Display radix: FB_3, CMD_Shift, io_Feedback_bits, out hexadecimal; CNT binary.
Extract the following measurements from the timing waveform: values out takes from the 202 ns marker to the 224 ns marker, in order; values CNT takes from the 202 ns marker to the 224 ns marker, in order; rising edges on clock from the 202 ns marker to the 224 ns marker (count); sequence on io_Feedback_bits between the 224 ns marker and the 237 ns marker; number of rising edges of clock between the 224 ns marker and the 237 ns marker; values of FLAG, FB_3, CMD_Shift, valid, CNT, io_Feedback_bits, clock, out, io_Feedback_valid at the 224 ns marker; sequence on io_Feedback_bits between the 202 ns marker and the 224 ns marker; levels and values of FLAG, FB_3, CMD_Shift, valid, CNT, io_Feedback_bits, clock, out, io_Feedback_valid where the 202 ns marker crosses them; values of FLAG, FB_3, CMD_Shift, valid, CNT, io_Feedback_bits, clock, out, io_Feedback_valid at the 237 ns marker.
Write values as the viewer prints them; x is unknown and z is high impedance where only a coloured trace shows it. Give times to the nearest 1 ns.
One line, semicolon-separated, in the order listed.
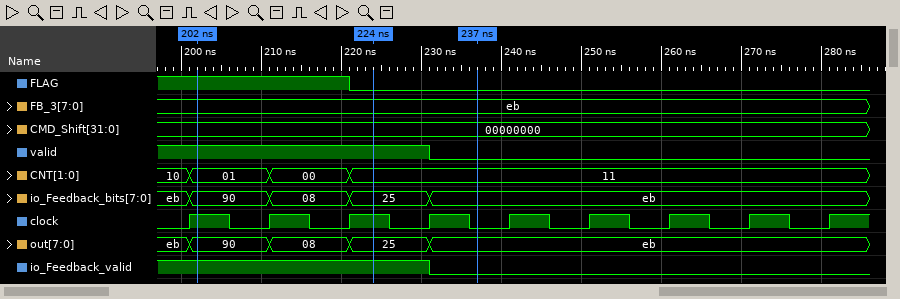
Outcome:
90, 08, 25; 01, 00, 11; 2; 25, eb; 1; FLAG=0, FB_3=eb, CMD_Shift=00000000, valid=1, CNT=11, io_Feedback_bits=25, clock=1, out=25, io_Feedback_valid=1; 90, 08, 25; FLAG=1, FB_3=eb, CMD_Shift=00000000, valid=1, CNT=01, io_Feedback_bits=90, clock=1, out=90, io_Feedback_valid=1; FLAG=0, FB_3=eb, CMD_Shift=00000000, valid=0, CNT=11, io_Feedback_bits=eb, clock=0, out=eb, io_Feedback_valid=0
